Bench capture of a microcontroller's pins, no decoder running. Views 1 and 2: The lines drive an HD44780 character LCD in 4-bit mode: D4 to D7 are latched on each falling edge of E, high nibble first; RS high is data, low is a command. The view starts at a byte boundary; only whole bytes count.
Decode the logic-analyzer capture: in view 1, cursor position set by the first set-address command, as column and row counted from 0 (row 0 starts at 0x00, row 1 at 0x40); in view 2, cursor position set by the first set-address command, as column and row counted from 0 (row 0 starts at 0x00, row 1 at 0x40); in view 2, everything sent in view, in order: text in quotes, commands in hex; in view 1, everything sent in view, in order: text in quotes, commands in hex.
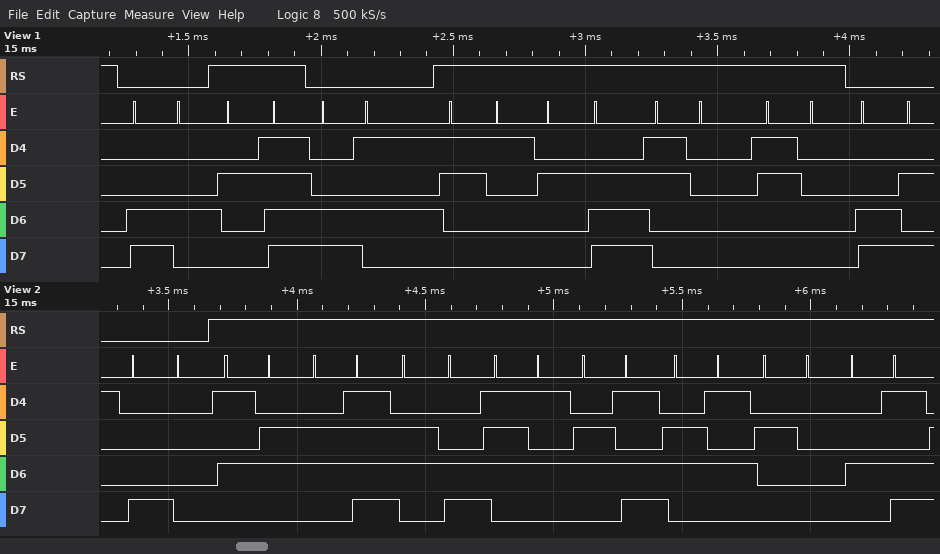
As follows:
column 4, row 1
column 0, row 0
0x80 "Volume M"
0xC4 "/" 0xC5 "1.00" 0xCA
